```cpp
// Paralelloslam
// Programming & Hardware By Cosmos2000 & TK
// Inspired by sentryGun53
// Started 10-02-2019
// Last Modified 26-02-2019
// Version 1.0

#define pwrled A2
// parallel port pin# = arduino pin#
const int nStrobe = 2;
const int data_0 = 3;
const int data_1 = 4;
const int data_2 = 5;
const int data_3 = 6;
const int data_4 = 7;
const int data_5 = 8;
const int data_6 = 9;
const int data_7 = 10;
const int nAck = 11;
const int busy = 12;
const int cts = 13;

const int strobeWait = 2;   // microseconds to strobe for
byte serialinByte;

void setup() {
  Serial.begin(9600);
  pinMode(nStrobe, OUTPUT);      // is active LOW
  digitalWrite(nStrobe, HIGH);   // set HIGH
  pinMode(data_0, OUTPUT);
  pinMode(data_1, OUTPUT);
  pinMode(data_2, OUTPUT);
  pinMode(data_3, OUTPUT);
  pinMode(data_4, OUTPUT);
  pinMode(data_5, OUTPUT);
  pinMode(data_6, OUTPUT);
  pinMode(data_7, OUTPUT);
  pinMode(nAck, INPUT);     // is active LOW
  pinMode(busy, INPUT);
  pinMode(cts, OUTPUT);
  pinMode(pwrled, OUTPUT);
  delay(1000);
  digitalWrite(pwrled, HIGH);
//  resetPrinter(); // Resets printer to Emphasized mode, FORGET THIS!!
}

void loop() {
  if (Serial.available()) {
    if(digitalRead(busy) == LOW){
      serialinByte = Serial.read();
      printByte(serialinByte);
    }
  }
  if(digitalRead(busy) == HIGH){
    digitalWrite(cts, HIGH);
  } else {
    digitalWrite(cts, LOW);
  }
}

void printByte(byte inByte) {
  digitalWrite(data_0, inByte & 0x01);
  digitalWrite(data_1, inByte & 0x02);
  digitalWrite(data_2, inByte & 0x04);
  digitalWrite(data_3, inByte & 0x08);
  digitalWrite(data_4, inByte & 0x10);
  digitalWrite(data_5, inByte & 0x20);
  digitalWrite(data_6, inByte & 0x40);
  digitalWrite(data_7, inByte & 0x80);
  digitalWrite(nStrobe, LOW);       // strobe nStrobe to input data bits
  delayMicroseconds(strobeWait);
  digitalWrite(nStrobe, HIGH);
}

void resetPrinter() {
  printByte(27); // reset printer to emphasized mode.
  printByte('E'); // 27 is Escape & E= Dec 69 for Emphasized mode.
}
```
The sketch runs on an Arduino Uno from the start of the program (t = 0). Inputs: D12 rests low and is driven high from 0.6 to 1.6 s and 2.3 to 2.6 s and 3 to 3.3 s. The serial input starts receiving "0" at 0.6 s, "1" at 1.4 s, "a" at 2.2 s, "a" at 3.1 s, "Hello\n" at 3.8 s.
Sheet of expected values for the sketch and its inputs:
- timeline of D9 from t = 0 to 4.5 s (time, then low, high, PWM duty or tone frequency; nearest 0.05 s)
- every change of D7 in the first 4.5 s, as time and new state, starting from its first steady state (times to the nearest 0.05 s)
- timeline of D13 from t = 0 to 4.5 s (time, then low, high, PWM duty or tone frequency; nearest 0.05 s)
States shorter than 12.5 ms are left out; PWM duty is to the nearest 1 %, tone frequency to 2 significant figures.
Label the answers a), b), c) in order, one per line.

a) 0 s low; 2.2 s high; 3.8 s low
b) 0 s low; 1.6 s high; 2.2 s low
c) 0 s low; 1 s high; 1.6 s low; 2.3 s high; 2.6 s low; 3 s high; 3.3 s low
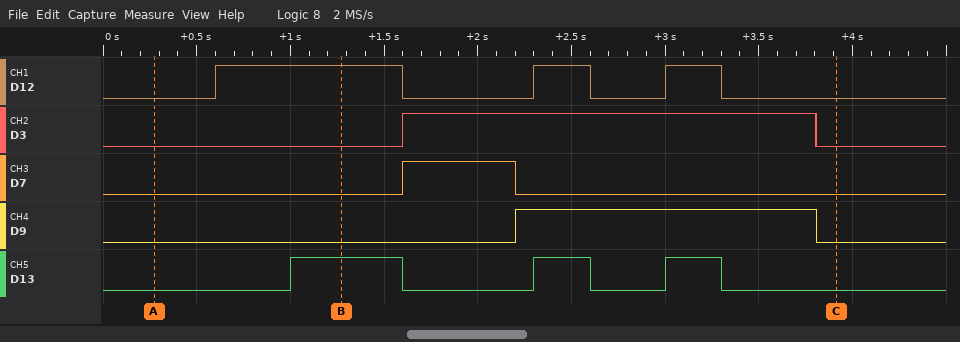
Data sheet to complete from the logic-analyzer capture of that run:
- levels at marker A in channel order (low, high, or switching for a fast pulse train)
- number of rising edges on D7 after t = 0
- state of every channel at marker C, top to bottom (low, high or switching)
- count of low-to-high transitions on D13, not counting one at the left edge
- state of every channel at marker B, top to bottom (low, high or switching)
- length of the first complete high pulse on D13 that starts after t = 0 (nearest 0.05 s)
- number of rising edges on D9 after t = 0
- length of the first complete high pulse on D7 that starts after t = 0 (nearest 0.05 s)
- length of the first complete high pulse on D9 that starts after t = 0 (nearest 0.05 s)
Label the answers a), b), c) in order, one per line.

a) D12 low, D3 low, D7 low, D9 low, D13 low
b) 1
c) D12 low, D3 low, D7 low, D9 low, D13 low
d) 3
e) D12 high, D3 low, D7 low, D9 low, D13 high
f) 0.60 s
g) 1
h) 0.60 s
i) 1.60 s
